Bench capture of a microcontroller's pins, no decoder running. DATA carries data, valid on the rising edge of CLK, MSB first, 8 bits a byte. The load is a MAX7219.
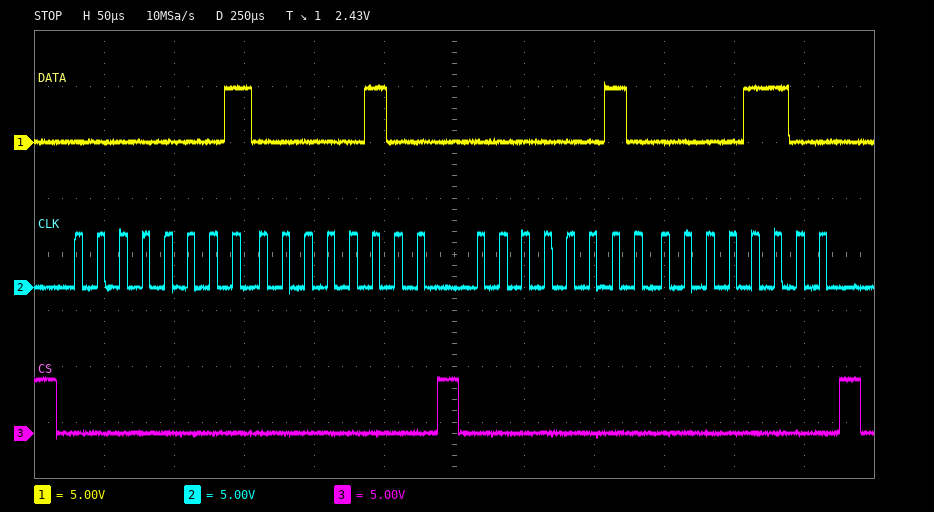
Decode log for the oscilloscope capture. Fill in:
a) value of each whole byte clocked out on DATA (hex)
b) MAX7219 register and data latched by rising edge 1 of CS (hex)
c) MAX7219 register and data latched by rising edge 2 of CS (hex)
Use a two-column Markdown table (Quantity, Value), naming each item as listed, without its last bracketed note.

| Quantity | Value |
|---|---|
| value of each whole byte clocked out on DATA | 01 04 02 0C |
| MAX7219 register and data latched by rising edge 1 of CS | register 0x1, data 0x04 |
| MAX7219 register and data latched by rising edge 2 of CS | register 0x2, data 0x0C |
